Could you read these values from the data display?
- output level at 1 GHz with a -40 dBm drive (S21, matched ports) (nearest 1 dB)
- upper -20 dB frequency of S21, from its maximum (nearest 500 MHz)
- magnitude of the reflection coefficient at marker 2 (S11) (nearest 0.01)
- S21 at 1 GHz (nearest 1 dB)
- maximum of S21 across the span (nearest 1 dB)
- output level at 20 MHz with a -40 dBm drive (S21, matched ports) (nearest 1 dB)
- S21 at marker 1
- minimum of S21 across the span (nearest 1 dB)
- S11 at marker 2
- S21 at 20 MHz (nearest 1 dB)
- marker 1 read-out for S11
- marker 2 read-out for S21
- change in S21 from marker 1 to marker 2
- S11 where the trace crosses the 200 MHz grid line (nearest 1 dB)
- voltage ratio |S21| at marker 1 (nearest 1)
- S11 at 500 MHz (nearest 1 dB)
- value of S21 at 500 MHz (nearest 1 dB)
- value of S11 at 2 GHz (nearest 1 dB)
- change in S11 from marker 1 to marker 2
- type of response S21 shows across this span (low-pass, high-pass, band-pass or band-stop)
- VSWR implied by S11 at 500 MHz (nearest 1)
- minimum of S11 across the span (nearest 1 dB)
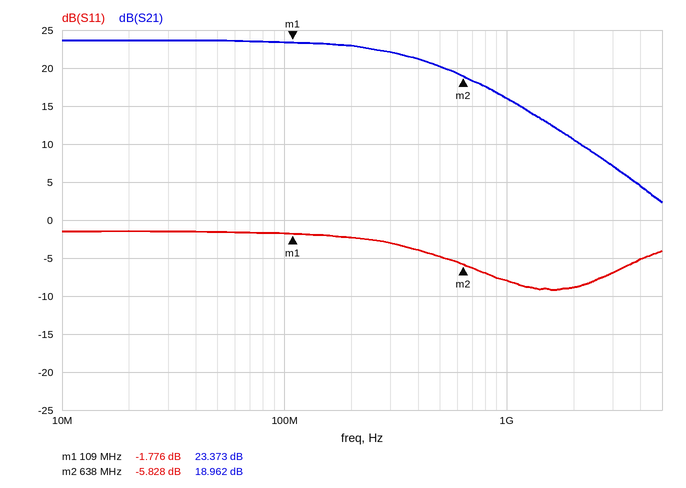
-24 dBm
4.5 GHz
0.51
16 dB
24 dB
-16 dBm
23.373 dB
2 dB
-5.828 dB
24 dB
-1.776 dB
18.962 dB
-4.411 dB
-2 dB
15
-5 dB
20 dB
-9 dB
-4.052 dB
low-pass
4
-9 dB
